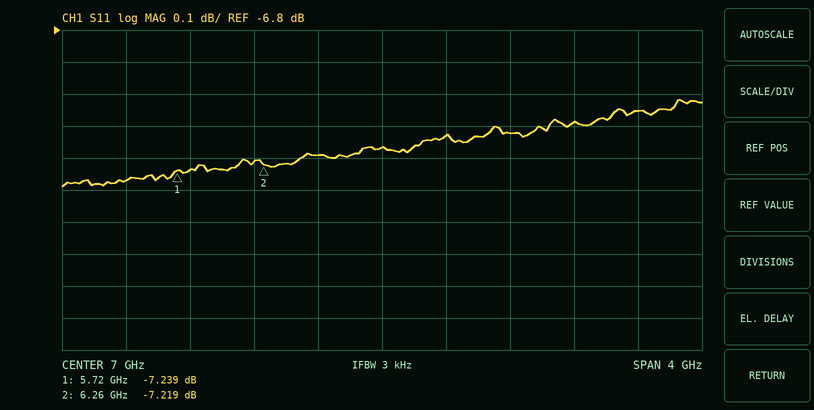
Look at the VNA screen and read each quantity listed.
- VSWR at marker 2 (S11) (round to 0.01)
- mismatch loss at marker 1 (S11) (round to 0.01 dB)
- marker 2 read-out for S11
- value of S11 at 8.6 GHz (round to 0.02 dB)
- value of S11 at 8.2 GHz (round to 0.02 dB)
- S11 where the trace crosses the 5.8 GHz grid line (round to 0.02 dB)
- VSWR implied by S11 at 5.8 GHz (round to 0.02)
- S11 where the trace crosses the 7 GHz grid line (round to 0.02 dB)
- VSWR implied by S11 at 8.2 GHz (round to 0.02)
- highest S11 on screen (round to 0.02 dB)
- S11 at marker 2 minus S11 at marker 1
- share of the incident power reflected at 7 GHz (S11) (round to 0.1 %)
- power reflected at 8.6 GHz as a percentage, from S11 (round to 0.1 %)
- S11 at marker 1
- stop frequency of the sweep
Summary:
2.54
0.91 dB
-7.219 dB
-7.06 dB
-7.08 dB
-7.24 dB
2.54
-7.16 dB
2.58
-7.02 dB
0.020 dB
19.2 %
19.7 %
-7.239 dB
9 GHz
